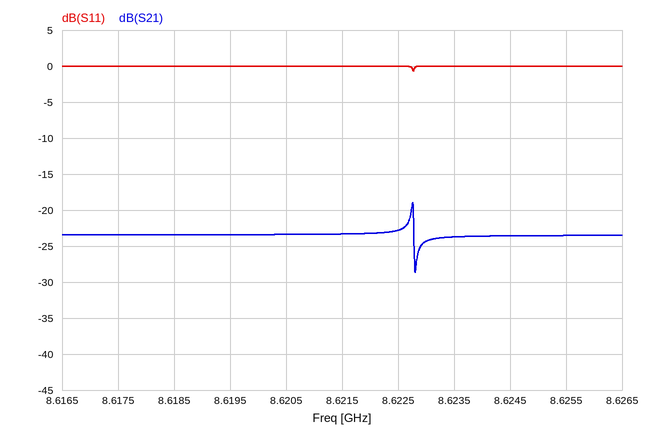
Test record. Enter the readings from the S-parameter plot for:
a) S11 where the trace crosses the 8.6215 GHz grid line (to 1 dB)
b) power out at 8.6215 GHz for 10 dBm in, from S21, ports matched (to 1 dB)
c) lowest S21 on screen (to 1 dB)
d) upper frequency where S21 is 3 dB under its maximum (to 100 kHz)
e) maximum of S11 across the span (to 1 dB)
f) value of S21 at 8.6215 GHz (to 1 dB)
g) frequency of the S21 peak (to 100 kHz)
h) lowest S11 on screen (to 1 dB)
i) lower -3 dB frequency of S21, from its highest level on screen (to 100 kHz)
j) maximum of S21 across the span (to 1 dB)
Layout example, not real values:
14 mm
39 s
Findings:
0 dB
-13 dBm
-29 dB
8.6228 GHz
0 dB
-23 dB
8.6228 GHz
-1 dB
8.6227 GHz
-19 dB
